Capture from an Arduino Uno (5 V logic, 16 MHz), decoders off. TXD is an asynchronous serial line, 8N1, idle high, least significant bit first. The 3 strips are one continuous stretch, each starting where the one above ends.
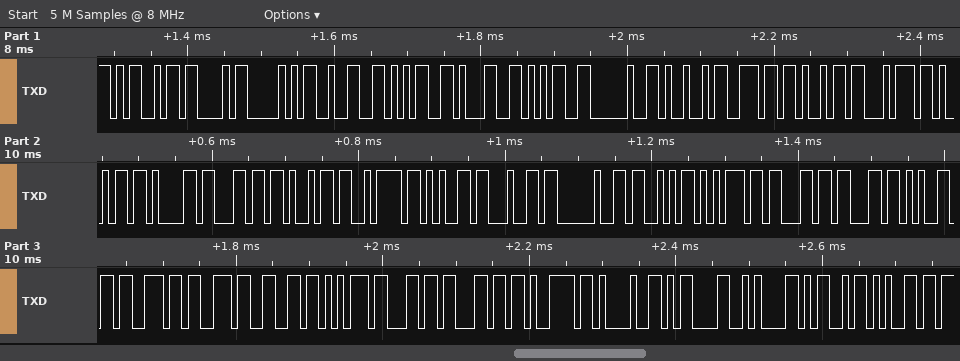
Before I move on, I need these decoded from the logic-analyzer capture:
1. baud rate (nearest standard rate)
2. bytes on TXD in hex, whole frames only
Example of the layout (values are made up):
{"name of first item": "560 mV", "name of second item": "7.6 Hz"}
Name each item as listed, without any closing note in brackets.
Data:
{"baud rate": "115200 baud", "bytes on TXD in hex, whole frames only": "0x4D 0x43 0x50 0x32 0x35 0x31 0x35 0x20 0x49 0x6E 0x69 0x74 0x69 0x61 0x6C 0x69 0x7A 0x65 0x64 0x20 0x53 0x75 0x63 0x63 0x65 0x73 0x73 0x66 0x75 0x6C 0x6C 0x79 0x21 0x0D 0x0A 0x4D 0x65"}
